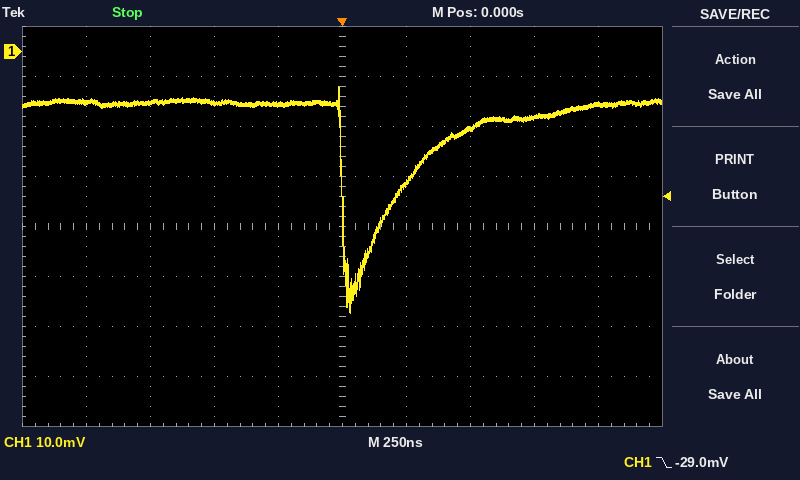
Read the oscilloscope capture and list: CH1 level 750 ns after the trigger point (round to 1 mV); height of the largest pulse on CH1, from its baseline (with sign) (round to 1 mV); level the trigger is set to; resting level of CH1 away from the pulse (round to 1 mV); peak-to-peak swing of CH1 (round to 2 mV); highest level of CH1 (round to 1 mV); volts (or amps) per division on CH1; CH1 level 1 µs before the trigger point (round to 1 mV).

-13 mV
-42 mV
-29.0 mV
-10 mV
46 mV
-7 mV
10 mV
-10 mV
